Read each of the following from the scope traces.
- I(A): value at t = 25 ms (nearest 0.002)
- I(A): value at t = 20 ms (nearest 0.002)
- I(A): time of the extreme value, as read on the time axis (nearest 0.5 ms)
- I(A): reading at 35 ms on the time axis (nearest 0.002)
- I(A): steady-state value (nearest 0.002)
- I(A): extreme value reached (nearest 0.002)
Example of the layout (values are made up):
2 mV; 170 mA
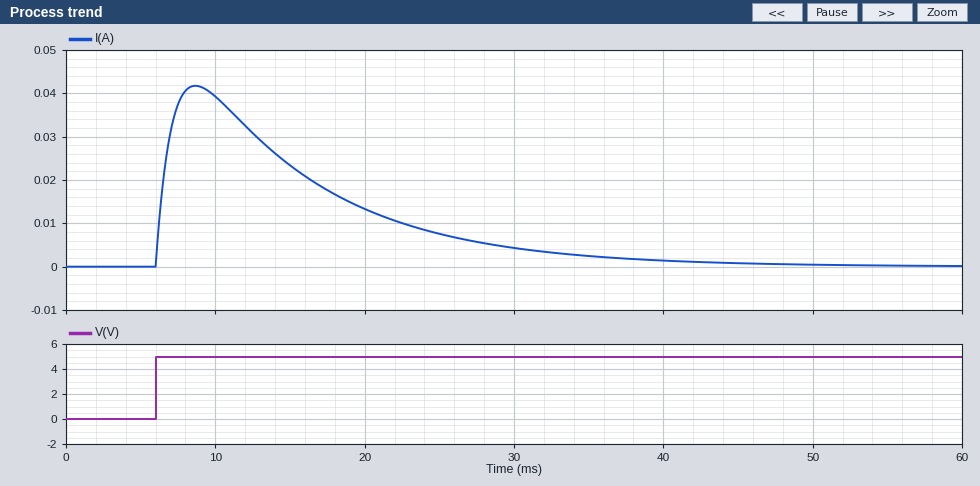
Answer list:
0.008; 0.014; 8.5 ms; 0.002; 0.000; 0.042
